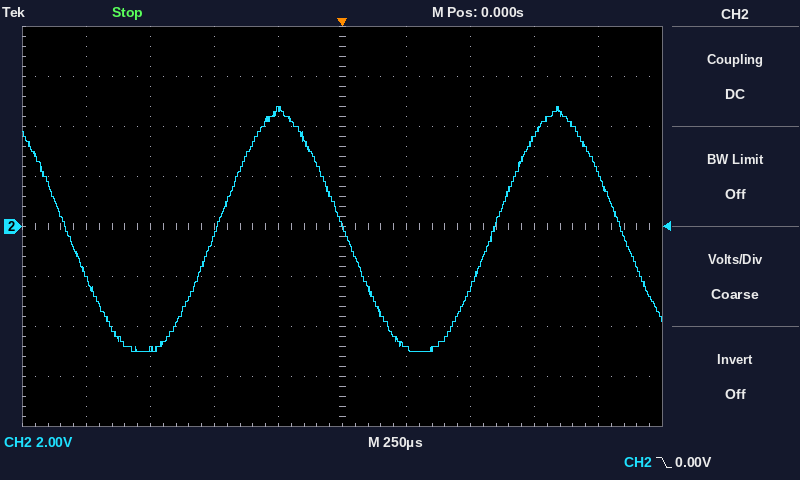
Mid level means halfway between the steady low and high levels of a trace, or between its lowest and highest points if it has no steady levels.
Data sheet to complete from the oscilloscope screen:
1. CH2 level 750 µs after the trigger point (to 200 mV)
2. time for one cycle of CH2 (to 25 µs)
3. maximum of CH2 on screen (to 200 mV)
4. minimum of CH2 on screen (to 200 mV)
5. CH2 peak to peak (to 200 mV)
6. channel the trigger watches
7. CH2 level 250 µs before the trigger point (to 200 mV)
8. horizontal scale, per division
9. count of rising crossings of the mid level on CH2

3.6 V
1.075 ms
4.8 V
-5.0 V
9.8 V
CH2
4.6 V
250 µs
2
